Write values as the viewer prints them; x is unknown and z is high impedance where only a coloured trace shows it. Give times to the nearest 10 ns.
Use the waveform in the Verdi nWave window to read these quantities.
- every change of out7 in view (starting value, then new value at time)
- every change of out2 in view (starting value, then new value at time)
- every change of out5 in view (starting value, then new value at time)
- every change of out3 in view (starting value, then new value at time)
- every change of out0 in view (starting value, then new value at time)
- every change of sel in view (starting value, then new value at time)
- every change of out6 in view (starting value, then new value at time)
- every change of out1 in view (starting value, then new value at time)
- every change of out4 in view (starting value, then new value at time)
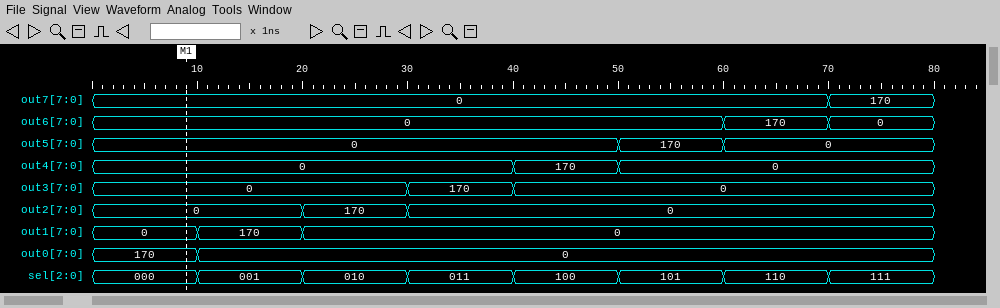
0, 170 at 70 ns
0, 170 at 20 ns, 0 at 30 ns
0, 170 at 50 ns, 0 at 60 ns
0, 170 at 30 ns, 0 at 40 ns
170, 0 at 10 ns
000, 001 at 10 ns, 010 at 20 ns, 011 at 30 ns, 100 at 40 ns, 101 at 50 ns, 110 at 60 ns, 111 at 70 ns
0, 170 at 60 ns, 0 at 70 ns
0, 170 at 10 ns, 0 at 20 ns
0, 170 at 40 ns, 0 at 50 ns
